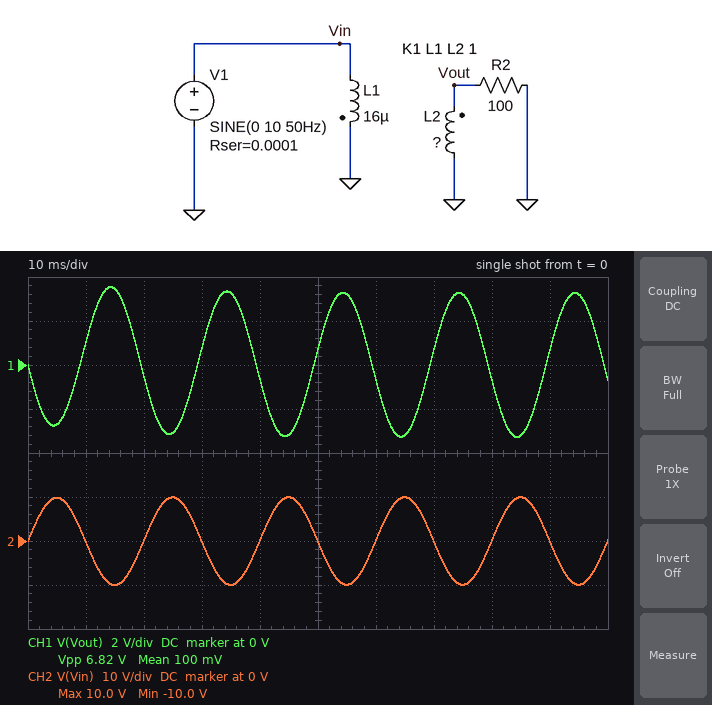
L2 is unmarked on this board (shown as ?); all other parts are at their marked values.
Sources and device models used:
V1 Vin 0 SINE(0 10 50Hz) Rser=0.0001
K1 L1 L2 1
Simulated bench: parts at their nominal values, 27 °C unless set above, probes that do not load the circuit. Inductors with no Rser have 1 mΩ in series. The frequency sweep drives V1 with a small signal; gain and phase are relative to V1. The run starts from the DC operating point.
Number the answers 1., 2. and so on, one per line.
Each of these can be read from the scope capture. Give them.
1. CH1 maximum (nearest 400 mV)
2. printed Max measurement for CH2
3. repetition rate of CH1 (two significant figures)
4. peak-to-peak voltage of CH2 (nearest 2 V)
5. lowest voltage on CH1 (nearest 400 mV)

1. 3.6 V
2. 10.0 V
3. 50 Hz
4. 20 V
5. -3.2 V
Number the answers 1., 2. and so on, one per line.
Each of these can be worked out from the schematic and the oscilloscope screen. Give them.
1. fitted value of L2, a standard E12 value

1. 1.8 µH
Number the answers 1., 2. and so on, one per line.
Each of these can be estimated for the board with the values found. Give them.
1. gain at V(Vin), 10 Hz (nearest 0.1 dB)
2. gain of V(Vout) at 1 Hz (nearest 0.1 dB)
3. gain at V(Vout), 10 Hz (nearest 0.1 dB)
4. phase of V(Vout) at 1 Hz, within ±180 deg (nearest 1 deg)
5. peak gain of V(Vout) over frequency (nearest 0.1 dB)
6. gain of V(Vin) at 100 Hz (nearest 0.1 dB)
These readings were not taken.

1. -0.4 dB
2. -30.3 dB
3. -12.9 dB
4. -95 deg
5. -9.5 dB
6. 0 dB
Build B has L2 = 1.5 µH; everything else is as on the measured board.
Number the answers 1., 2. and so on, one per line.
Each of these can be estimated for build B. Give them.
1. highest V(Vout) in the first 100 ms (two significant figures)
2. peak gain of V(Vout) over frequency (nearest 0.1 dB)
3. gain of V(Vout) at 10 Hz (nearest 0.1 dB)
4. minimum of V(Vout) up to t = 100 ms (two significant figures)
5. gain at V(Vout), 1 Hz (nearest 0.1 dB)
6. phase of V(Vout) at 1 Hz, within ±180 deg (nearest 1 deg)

1. 3.2 V
2. -10.3 dB
3. -13.7 dB
4. -3.0 V
5. -31.1 dB
6. -95 deg
